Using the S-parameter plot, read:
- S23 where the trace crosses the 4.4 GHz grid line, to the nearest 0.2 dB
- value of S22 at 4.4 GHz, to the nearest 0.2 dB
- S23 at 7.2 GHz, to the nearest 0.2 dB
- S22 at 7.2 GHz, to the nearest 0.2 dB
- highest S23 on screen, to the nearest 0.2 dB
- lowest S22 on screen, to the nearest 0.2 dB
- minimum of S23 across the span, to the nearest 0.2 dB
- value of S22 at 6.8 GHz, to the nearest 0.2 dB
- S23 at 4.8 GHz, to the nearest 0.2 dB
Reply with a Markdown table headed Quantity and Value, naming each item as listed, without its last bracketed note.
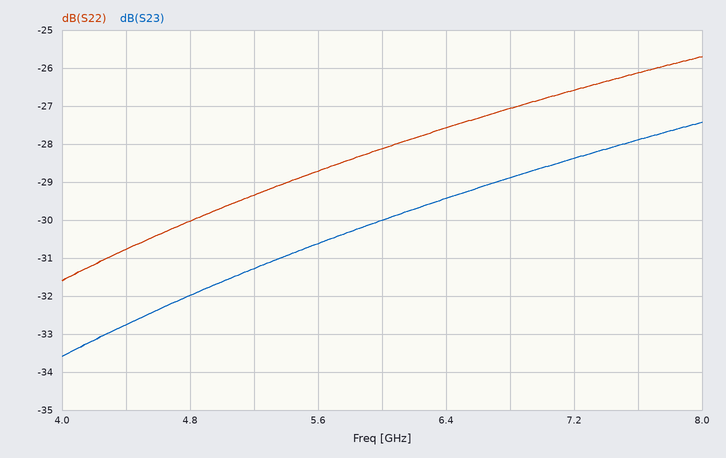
| Quantity | Value |
|---|---|
| S23 where the trace crosses the 4.4 GHz grid line, to the nearest 0.2 dB | -32.8 dB |
| value of S22 at 4.4 GHz, to the nearest 0.2 dB | -30.8 dB |
| S23 at 7.2 GHz, to the nearest 0.2 dB | -28.4 dB |
| S22 at 7.2 GHz, to the nearest 0.2 dB | -26.6 dB |
| highest S23 on screen, to the nearest 0.2 dB | -27.4 dB |
| lowest S22 on screen, to the nearest 0.2 dB | -31.6 dB |
| minimum of S23 across the span, to the nearest 0.2 dB | -33.6 dB |
| value of S22 at 6.8 GHz, to the nearest 0.2 dB | -27.0 dB |
| S23 at 4.8 GHz, to the nearest 0.2 dB | -32.0 dB |
